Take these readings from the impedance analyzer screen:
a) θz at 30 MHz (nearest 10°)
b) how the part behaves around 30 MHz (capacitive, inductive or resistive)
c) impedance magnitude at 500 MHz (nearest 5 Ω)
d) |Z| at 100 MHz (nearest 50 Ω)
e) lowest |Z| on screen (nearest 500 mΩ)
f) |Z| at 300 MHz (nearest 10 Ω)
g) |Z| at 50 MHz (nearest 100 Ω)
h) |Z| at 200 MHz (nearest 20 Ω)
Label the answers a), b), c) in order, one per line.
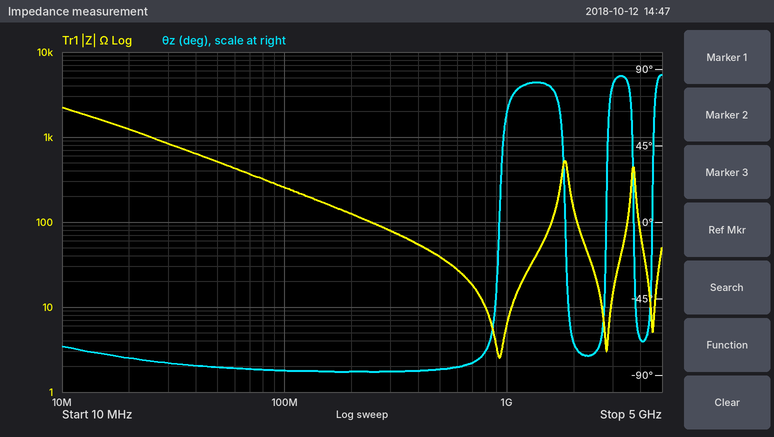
a) -80°
b) capacitive
c) 40 Ω
d) 250 Ω
e) 2.5 Ω
f) 80 Ω
g) 500 Ω
h) 120 Ω
